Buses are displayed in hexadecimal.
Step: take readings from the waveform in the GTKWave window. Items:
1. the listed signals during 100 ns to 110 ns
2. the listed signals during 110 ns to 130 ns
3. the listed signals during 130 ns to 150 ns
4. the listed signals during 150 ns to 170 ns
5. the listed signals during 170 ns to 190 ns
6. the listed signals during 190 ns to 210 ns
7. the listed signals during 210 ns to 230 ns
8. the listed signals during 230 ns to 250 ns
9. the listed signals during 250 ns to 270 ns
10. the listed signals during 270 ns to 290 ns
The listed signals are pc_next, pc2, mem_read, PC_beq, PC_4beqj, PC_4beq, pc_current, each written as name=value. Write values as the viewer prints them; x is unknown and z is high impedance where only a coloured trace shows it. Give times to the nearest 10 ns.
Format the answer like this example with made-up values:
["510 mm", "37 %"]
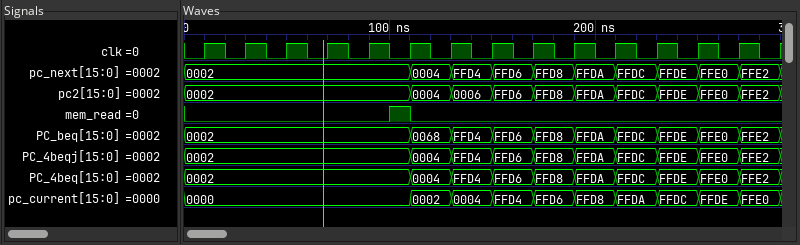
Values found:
["pc_next=0002, pc2=0002, mem_read=1, PC_beq=0002, PC_4beqj=0002, PC_4beq=0002, pc_current=0000", "pc_next=0004, pc2=0004, mem_read=0, PC_beq=0068, PC_4beqj=0004, PC_4beq=0004, pc_current=0002", "pc_next=FFD4, pc2=0006, mem_read=0, PC_beq=FFD4, PC_4beqj=FFD4, PC_4beq=FFD4, pc_current=0004", "pc_next=FFD6, pc2=FFD6, mem_read=0, PC_beq=FFD6, PC_4beqj=FFD6, PC_4beq=FFD6, pc_current=FFD4", "pc_next=FFD8, pc2=FFD8, mem_read=0, PC_beq=FFD8, PC_4beqj=FFD8, PC_4beq=FFD8, pc_current=FFD6", "pc_next=FFDA, pc2=FFDA, mem_read=0, PC_beq=FFDA, PC_4beqj=FFDA, PC_4beq=FFDA, pc_current=FFD8", "pc_next=FFDC, pc2=FFDC, mem_read=0, PC_beq=FFDC, PC_4beqj=FFDC, PC_4beq=FFDC, pc_current=FFDA", "pc_next=FFDE, pc2=FFDE, mem_read=0, PC_beq=FFDE, PC_4beqj=FFDE, PC_4beq=FFDE, pc_current=FFDC", "pc_next=FFE0, pc2=FFE0, mem_read=0, PC_beq=FFE0, PC_4beqj=FFE0, PC_4beq=FFE0, pc_current=FFDE", "pc_next=FFE2, pc2=FFE2, mem_read=0, PC_beq=FFE2, PC_4beqj=FFE2, PC_4beq=FFE2, pc_current=FFE0"]
